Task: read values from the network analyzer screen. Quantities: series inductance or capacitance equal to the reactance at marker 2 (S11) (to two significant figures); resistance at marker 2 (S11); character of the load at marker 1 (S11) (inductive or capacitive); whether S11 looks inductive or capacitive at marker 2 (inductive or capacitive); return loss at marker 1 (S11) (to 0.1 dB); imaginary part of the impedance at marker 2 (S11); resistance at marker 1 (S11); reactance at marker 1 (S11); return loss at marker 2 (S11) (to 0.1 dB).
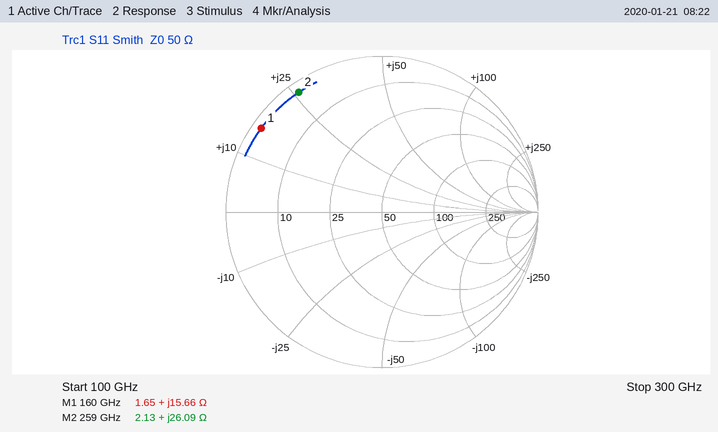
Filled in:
16 pH
2.13 Ω
inductive
inductive
0.5 dB
+26.09 Ω
1.65 Ω
+15.66 Ω
0.6 dB
